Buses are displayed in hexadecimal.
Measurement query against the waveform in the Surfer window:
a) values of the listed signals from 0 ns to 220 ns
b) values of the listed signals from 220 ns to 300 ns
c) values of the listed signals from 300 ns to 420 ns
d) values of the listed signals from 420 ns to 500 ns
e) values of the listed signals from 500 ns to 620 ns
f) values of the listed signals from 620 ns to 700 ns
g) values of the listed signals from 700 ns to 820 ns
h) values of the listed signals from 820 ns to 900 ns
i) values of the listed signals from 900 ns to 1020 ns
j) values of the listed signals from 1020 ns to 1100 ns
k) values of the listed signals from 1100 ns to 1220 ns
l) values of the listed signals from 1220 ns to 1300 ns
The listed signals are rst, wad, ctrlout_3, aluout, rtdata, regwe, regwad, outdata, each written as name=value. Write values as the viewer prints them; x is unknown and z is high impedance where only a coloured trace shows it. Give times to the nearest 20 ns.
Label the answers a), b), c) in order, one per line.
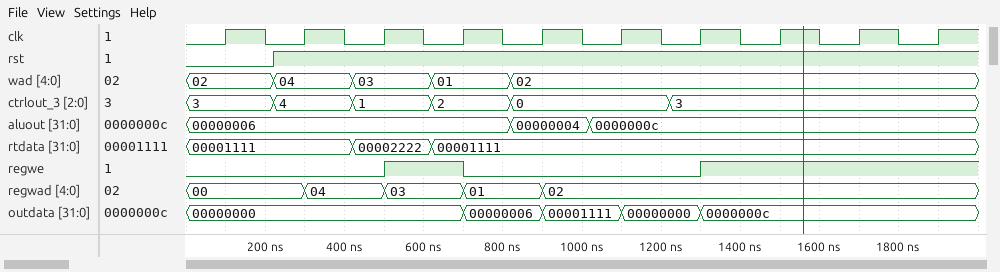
a) rst=0, wad=02, ctrlout_3=3, aluout=00000006, rtdata=00001111, regwe=0, regwad=00, outdata=00000000
b) rst=1, wad=04, ctrlout_3=4, aluout=00000006, rtdata=00001111, regwe=0, regwad=00, outdata=00000000
c) rst=1, wad=04, ctrlout_3=4, aluout=00000006, rtdata=00001111, regwe=0, regwad=04, outdata=00000000
d) rst=1, wad=03, ctrlout_3=1, aluout=00000006, rtdata=00002222, regwe=0, regwad=04, outdata=00000000
e) rst=1, wad=03, ctrlout_3=1, aluout=00000006, rtdata=00002222, regwe=1, regwad=03, outdata=00000000
f) rst=1, wad=01, ctrlout_3=2, aluout=00000006, rtdata=00001111, regwe=1, regwad=03, outdata=00000000
g) rst=1, wad=01, ctrlout_3=2, aluout=00000006, rtdata=00001111, regwe=0, regwad=01, outdata=00000006
h) rst=1, wad=02, ctrlout_3=0, aluout=00000004, rtdata=00001111, regwe=0, regwad=01, outdata=00000006
i) rst=1, wad=02, ctrlout_3=0, aluout=00000004, rtdata=00001111, regwe=0, regwad=02, outdata=00001111
j) rst=1, wad=02, ctrlout_3=0, aluout=0000000c, rtdata=00001111, regwe=0, regwad=02, outdata=00001111
k) rst=1, wad=02, ctrlout_3=0, aluout=0000000c, rtdata=00001111, regwe=0, regwad=02, outdata=00000000
l) rst=1, wad=02, ctrlout_3=3, aluout=0000000c, rtdata=00001111, regwe=0, regwad=02, outdata=00000000
